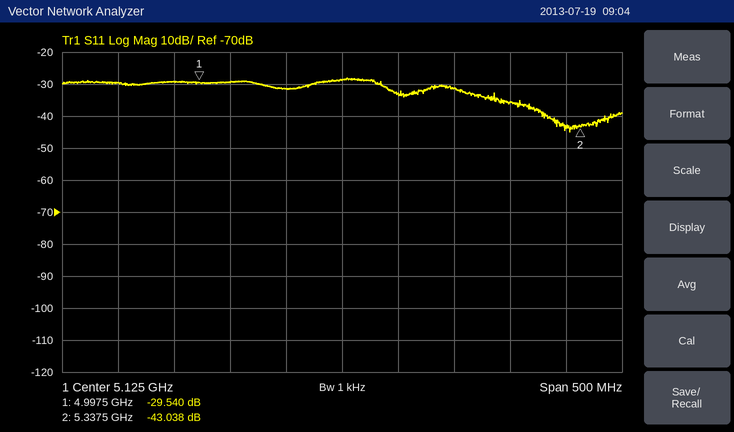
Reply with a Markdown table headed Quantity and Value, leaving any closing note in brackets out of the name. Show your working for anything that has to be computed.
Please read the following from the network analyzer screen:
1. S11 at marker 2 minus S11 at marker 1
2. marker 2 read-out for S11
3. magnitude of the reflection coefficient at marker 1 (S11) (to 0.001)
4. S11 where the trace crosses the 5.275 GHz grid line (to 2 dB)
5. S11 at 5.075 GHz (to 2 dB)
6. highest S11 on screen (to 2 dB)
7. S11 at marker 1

| Quantity | Value |
|---|---|
| S11 at marker 2 minus S11 at marker 1 | -43.038 − (-29.54) = -13.498 dB |
| marker 2 read-out for S11 | -43.038 dB |
| magnitude of the reflection coefficient at marker 1 (S11) | 10^(-29.54/20) ≈ 0.033 |
| S11 where the trace crosses the 5.275 GHz grid line | -36 dB |
| S11 at 5.075 GHz | -32 dB |
| highest S11 on screen | -28 dB |
| S11 at marker 1 | -29.540 dB |
